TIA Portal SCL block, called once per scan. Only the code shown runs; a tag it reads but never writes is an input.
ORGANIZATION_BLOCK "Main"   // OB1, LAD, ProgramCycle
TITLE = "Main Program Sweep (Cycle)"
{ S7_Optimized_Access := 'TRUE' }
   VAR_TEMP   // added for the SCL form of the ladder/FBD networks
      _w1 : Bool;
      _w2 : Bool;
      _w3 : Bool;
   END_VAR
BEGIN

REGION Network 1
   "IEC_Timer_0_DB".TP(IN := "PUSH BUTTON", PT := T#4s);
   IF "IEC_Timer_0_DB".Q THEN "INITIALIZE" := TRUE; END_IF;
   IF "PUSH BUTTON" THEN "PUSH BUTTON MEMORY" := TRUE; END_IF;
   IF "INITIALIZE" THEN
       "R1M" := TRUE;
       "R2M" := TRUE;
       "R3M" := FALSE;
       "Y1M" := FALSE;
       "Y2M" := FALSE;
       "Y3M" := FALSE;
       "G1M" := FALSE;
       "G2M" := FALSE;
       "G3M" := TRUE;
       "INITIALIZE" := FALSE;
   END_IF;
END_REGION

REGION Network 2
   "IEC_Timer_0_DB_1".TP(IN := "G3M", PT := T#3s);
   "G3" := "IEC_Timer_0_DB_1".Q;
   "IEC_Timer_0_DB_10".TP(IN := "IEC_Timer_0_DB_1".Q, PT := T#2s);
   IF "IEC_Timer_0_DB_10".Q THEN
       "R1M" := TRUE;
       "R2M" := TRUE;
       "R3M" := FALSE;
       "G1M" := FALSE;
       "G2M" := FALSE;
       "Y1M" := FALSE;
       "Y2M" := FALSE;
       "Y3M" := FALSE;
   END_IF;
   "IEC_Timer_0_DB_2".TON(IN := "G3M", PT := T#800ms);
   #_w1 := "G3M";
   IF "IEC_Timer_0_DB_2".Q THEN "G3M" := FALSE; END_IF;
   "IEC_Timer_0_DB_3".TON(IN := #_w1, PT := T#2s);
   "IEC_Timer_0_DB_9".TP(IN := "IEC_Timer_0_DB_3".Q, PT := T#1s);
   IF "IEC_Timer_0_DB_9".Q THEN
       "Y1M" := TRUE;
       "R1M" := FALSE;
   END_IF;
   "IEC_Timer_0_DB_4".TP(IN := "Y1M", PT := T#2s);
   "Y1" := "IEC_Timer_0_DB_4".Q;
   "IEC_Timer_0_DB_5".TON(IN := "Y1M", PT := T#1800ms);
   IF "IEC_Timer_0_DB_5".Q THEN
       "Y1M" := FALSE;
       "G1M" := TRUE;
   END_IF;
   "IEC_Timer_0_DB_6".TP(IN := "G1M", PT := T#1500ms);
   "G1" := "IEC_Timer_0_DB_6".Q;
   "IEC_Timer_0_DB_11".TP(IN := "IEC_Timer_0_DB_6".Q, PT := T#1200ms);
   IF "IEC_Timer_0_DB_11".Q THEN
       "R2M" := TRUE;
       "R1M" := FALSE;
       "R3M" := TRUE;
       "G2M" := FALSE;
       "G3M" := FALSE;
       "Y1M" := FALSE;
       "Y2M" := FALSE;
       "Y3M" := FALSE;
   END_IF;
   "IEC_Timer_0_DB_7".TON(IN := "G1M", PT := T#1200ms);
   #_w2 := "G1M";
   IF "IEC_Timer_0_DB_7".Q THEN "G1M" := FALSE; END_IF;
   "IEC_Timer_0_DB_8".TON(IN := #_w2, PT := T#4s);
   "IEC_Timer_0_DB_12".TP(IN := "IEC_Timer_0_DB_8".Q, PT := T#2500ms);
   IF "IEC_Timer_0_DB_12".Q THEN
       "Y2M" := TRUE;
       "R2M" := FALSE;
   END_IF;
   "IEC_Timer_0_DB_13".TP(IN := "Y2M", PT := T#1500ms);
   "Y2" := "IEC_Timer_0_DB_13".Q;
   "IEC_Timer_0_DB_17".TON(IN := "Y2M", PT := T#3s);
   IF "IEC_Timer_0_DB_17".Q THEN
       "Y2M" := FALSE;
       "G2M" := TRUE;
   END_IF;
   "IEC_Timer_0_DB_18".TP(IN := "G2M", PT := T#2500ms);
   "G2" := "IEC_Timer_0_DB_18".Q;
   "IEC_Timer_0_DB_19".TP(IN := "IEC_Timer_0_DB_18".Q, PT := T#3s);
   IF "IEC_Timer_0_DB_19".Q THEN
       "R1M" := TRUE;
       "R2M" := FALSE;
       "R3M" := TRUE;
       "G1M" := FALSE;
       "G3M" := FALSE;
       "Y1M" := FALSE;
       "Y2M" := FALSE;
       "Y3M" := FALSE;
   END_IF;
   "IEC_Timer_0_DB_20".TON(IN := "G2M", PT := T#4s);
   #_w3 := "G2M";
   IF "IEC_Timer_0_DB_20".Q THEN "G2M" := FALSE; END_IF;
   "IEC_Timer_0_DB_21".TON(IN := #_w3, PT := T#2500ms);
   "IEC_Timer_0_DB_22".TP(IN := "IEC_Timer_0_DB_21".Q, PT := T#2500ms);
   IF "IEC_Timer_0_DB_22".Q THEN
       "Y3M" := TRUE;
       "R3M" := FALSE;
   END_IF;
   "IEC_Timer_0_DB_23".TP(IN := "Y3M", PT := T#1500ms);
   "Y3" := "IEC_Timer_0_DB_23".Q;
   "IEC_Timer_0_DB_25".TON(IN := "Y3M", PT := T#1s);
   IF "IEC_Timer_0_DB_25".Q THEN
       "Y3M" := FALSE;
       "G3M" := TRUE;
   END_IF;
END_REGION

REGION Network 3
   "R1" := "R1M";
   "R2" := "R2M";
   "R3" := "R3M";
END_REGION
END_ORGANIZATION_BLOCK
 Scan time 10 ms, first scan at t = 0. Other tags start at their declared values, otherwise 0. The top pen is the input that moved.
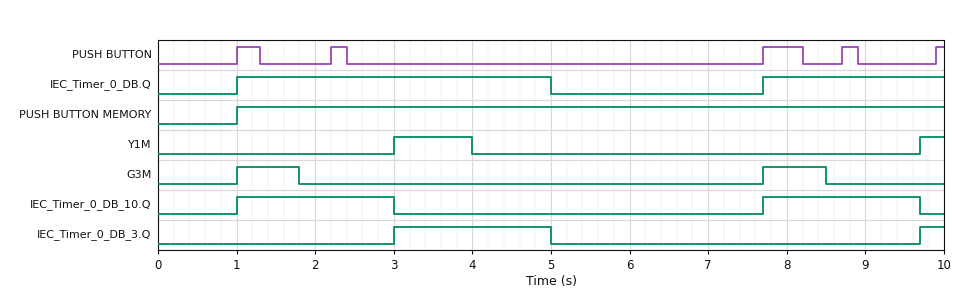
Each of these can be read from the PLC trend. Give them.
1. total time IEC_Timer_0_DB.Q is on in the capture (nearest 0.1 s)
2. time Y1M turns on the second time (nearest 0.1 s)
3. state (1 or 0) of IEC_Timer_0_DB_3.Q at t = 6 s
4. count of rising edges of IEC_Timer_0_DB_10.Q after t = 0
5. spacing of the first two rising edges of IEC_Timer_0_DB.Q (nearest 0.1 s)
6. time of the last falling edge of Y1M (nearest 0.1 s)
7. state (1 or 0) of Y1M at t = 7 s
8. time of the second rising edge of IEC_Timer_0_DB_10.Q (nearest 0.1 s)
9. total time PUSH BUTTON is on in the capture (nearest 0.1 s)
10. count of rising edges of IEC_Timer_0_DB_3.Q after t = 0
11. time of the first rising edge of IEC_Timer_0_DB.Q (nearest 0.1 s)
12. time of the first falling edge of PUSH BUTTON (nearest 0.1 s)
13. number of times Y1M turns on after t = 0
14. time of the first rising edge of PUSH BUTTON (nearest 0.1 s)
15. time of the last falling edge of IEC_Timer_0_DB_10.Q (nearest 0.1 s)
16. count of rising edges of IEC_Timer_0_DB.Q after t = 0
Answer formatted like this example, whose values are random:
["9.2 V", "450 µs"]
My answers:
["6.3 s", "9.7 s", "0", "2", "6.7 s", "4.0 s", "0", "7.7 s", "1.3 s", "2", "1.0 s", "1.3 s", "2", "1.0 s", "9.7 s", "2"]
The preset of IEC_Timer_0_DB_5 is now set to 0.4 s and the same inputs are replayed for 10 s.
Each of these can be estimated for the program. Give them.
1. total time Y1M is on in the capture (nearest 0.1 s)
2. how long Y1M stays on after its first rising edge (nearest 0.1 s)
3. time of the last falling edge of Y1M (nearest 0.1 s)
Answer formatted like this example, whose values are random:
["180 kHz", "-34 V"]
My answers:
["0.7 s", "0.4 s", "3.4 s"]
